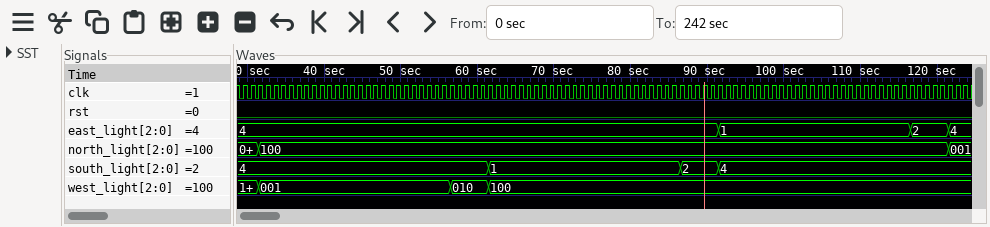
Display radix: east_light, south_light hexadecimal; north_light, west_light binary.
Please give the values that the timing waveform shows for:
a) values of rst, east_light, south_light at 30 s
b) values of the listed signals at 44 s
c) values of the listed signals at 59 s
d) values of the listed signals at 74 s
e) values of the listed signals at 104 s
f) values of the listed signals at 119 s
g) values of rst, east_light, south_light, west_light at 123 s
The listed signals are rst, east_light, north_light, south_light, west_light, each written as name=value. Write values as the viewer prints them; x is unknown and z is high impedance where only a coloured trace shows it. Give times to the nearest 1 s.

rst=0, east_light=4, south_light=4
rst=0, east_light=4, north_light=100, south_light=4, west_light=001
rst=0, east_light=4, north_light=100, south_light=4, west_light=010
rst=0, east_light=4, north_light=100, south_light=1, west_light=100
rst=0, east_light=1, north_light=100, south_light=4, west_light=100
rst=0, east_light=2, north_light=100, south_light=4, west_light=100
rst=0, east_light=4, south_light=4, west_light=100
